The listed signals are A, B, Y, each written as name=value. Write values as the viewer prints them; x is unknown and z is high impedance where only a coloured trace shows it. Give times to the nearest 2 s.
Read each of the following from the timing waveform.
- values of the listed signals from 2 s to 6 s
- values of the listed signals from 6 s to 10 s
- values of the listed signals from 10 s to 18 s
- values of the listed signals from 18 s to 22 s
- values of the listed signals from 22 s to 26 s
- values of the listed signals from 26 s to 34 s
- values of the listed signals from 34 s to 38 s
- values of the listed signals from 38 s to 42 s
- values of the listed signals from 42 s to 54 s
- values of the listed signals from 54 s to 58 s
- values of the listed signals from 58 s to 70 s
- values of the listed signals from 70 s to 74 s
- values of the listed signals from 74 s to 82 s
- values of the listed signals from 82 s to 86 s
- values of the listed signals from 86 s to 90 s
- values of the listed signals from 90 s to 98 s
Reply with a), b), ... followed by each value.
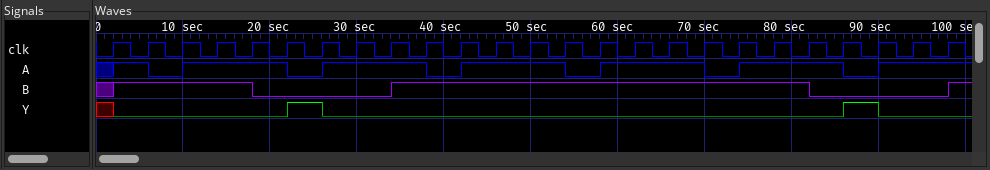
a) A=1, B=1, Y=0
b) A=0, B=1, Y=0
c) A=1, B=1, Y=0
d) A=1, B=0, Y=0
e) A=0, B=0, Y=1
f) A=1, B=0, Y=0
g) A=1, B=1, Y=0
h) A=0, B=1, Y=0
i) A=1, B=1, Y=0
j) A=0, B=1, Y=0
k) A=1, B=1, Y=0
l) A=0, B=1, Y=0
m) A=1, B=1, Y=0
n) A=1, B=0, Y=0
o) A=0, B=0, Y=1
p) A=1, B=0, Y=0
